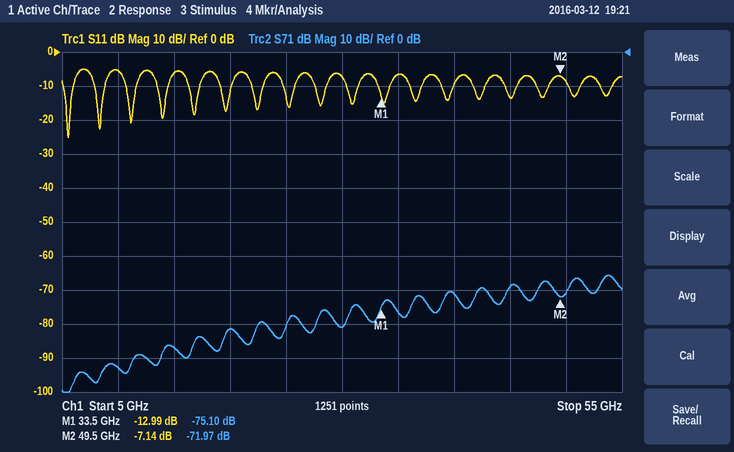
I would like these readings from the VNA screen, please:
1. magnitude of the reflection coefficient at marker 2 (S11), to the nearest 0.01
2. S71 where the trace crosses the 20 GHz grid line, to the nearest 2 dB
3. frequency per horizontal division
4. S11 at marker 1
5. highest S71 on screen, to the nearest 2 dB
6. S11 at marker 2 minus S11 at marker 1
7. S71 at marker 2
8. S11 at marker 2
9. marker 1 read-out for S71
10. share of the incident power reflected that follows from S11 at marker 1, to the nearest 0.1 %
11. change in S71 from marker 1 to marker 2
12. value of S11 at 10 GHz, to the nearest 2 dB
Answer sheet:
0.44
-82 dB
5 GHz
-12.99 dB
-66 dB
5.85 dB
-71.97 dB
-7.14 dB
-75.10 dB
5.0 %
3.13 dB
-6 dB
